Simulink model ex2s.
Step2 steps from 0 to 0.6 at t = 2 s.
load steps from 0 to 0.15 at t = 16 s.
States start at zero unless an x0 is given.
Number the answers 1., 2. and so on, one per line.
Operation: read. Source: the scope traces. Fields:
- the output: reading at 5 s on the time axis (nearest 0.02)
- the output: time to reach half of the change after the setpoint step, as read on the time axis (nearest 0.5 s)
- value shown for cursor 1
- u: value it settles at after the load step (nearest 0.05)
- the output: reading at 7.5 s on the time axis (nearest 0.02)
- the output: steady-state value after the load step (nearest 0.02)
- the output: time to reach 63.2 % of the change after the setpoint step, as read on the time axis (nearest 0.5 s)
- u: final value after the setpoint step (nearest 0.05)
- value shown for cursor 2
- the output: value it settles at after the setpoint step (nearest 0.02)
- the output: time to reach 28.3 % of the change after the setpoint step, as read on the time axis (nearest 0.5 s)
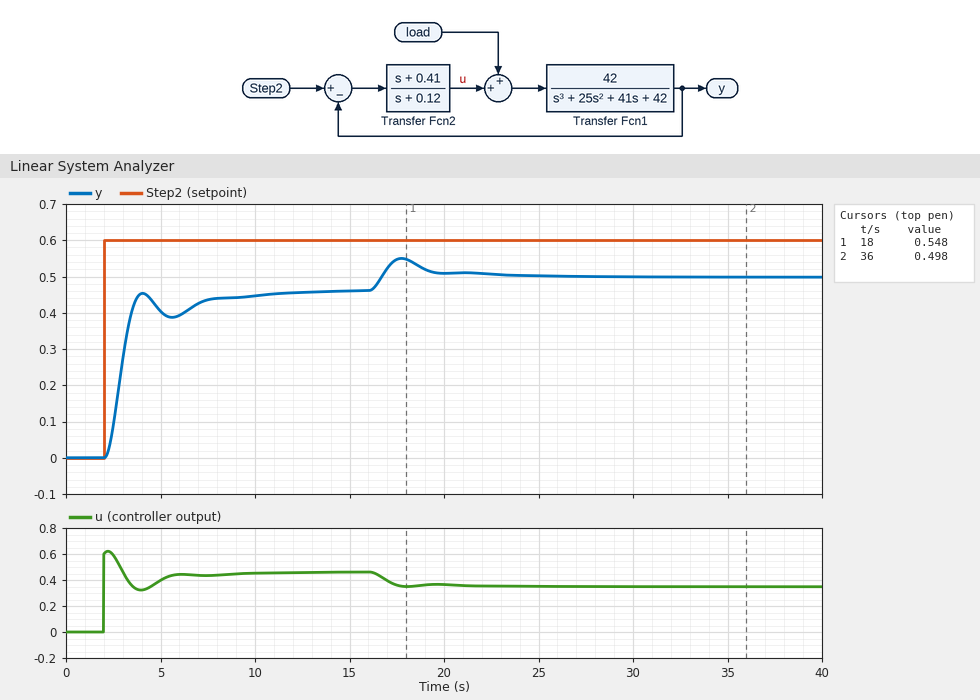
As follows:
1. 0.40
2. 3.0 s
3. 0.548
4. 0.35
5. 0.44
6. 0.50
7. 3.0 s
8. 0.45
9. 0.498
10. 0.46
11. 2.5 s
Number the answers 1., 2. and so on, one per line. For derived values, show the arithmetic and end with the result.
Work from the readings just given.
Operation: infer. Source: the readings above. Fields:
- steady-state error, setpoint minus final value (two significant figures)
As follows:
1. 0.6 - 0.46 = 0.14
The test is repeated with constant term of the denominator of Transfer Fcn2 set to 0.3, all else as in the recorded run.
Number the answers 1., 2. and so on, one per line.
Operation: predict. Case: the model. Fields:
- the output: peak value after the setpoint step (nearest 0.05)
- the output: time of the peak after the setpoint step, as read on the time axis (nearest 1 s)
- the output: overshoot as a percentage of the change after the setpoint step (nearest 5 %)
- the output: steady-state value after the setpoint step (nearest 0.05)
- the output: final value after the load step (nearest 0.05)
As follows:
1. 0.40
2. 4 s
3. 15 %
4. 0.35
5. 0.40
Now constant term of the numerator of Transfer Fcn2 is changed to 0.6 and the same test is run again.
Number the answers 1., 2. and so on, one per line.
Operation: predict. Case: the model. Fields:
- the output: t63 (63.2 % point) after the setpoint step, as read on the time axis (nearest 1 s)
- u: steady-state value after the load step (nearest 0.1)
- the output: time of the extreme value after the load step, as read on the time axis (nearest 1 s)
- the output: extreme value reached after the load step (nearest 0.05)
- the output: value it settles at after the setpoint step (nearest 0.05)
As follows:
1. 3 s
2. 0.4
3. 18 s
4. 0.60
5. 0.50
